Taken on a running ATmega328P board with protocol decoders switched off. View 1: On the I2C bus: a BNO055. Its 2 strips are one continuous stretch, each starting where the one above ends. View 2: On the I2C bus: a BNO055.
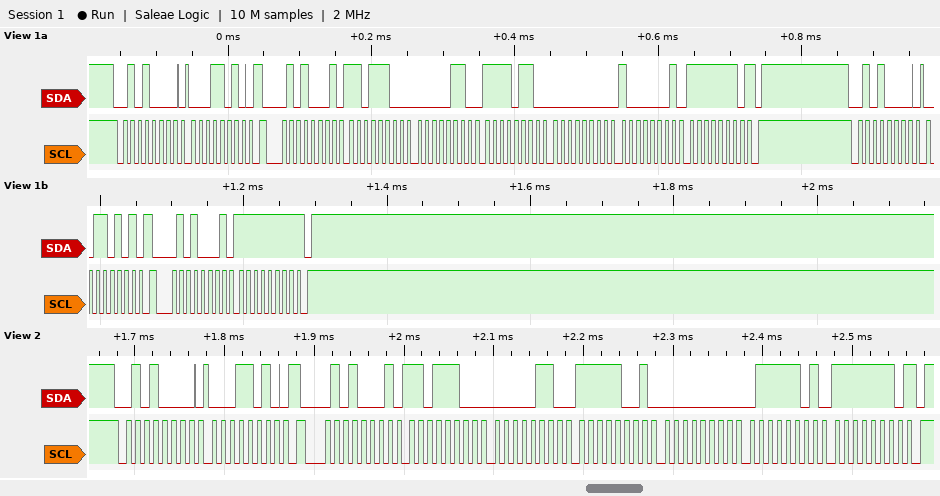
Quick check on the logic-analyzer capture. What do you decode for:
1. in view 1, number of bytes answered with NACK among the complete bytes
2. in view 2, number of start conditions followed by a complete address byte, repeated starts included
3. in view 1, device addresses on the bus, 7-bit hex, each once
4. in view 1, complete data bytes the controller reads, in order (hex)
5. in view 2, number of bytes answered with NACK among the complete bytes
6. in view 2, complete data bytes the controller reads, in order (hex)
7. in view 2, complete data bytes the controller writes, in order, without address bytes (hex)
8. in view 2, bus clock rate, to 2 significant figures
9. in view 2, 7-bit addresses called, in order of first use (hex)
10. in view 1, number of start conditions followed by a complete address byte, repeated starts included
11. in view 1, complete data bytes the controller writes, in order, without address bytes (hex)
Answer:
2
2
0x28
DC 06 F6 00 81 FE FF
1
DC 06 F9 00 7D FE
1A
100 kHz
0x28
4
1A 35
